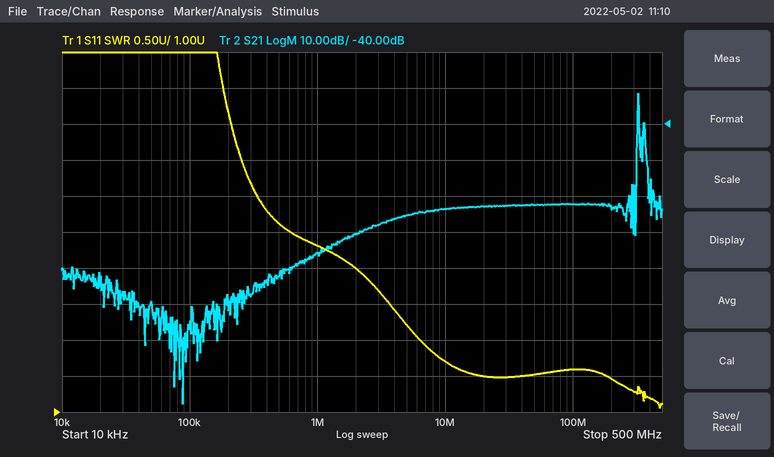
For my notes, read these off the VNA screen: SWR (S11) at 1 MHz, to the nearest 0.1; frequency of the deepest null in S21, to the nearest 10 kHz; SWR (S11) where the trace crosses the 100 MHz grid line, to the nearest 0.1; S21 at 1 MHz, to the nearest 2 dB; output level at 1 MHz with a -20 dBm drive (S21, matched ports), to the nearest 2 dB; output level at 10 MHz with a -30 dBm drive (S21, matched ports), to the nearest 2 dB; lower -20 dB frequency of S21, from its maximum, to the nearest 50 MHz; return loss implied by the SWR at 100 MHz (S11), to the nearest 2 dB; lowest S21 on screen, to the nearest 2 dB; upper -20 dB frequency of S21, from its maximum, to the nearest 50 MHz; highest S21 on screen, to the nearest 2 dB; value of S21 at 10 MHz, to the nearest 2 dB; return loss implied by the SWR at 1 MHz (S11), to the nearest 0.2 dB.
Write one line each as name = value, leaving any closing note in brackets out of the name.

SWR (S11) at 1 MHz, to the nearest 0.1 = 3.3
frequency of the deepest null in S21, to the nearest 10 kHz = 90 kHz
SWR (S11) where the trace crosses the 100 MHz grid line, to the nearest 0.1 = 1.6
S21 at 1 MHz, to the nearest 2 dB = -76 dB
output level at 1 MHz with a -20 dBm drive (S21, matched ports), to the nearest 2 dB = -96 dBm
output level at 10 MHz with a -30 dBm drive (S21, matched ports), to the nearest 2 dB = -94 dBm
lower -20 dB frequency of S21, from its maximum, to the nearest 50 MHz = 300 MHz
return loss implied by the SWR at 100 MHz (S11), to the nearest 2 dB = 12 dB
lowest S21 on screen, to the nearest 2 dB = -118 dB
upper -20 dB frequency of S21, from its maximum, to the nearest 50 MHz = 400 MHz
highest S21 on screen, to the nearest 2 dB = -32 dB
value of S21 at 10 MHz, to the nearest 2 dB = -64 dB
return loss implied by the SWR at 1 MHz (S11), to the nearest 0.2 dB = 5.4 dB
